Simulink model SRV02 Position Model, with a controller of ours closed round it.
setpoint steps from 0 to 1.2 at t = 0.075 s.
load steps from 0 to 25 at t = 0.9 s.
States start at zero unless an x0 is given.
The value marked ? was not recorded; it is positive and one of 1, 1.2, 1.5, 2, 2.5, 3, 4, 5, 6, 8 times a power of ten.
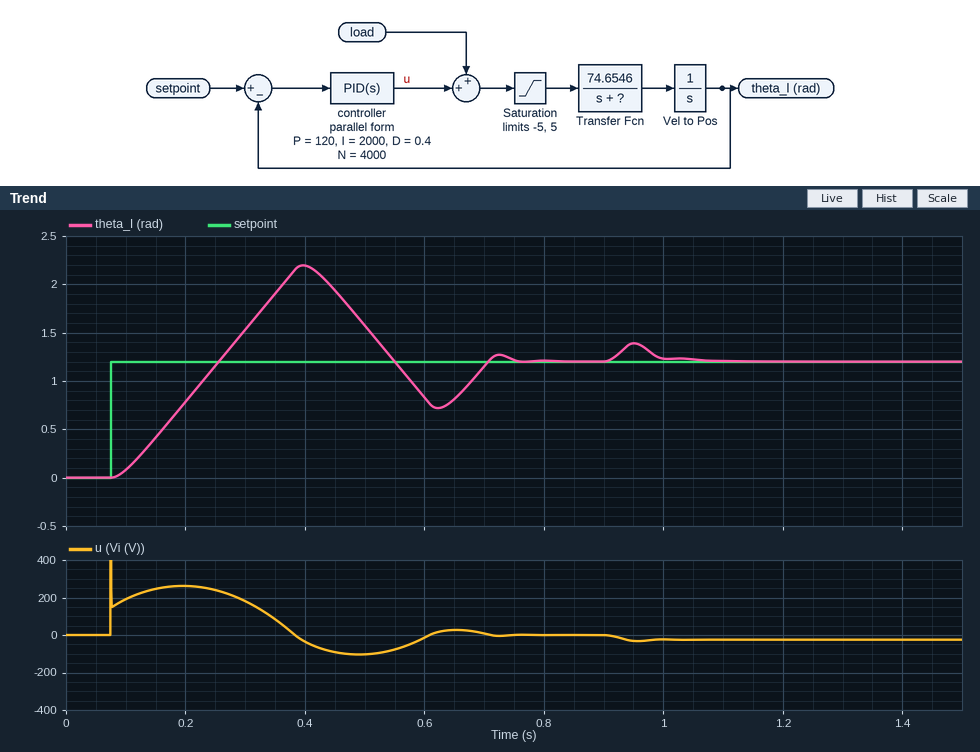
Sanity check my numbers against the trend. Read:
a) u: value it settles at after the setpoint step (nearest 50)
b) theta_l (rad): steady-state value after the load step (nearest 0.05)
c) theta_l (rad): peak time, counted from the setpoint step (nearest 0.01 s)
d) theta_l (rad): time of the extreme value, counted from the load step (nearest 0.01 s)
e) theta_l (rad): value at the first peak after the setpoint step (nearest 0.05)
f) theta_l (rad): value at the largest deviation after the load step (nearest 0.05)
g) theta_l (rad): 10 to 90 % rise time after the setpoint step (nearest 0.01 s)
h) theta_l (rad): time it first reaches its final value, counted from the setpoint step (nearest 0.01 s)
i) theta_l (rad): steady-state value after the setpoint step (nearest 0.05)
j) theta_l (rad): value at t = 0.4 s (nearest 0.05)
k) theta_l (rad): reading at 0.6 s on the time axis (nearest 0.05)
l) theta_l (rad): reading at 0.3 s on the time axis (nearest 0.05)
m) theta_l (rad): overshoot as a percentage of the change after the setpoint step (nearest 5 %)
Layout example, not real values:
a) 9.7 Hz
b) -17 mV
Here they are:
a) 0
b) 1.20
c) 0.32 s
d) 0.05 s
e) 2.20
f) 1.40
g) 0.13 s
h) 0.18 s
i) 1.20
j) 2.20
k) 0.85
l) 1.55
m) 85 %
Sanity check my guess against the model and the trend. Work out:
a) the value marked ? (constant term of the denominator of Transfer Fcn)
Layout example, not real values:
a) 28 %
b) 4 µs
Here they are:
a) 50
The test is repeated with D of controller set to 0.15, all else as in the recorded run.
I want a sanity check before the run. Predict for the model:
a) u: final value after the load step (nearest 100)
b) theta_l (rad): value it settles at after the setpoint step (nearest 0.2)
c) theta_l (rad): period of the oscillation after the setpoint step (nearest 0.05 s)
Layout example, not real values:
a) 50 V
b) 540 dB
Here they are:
a) 0
b) 1.2
c) 0.35 s
